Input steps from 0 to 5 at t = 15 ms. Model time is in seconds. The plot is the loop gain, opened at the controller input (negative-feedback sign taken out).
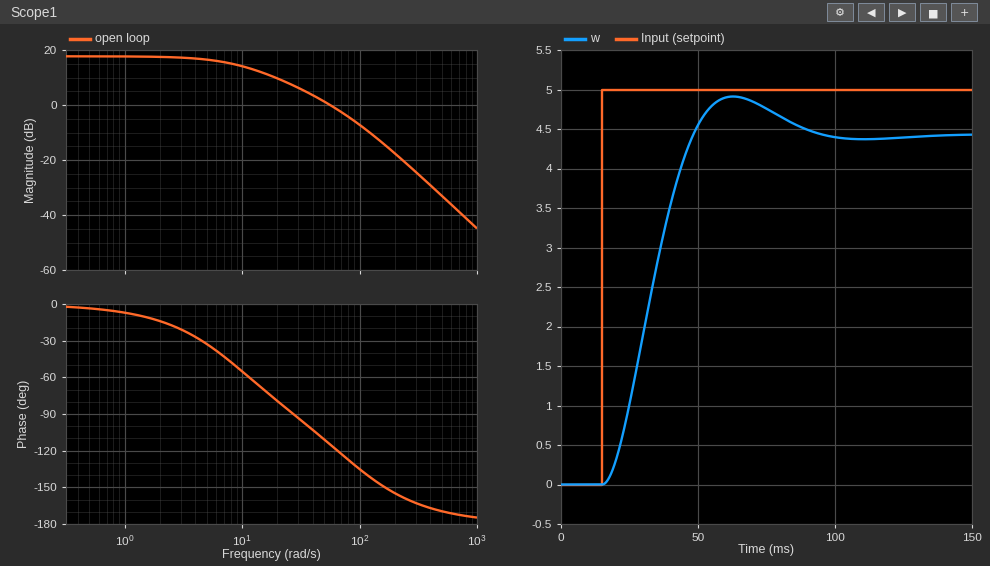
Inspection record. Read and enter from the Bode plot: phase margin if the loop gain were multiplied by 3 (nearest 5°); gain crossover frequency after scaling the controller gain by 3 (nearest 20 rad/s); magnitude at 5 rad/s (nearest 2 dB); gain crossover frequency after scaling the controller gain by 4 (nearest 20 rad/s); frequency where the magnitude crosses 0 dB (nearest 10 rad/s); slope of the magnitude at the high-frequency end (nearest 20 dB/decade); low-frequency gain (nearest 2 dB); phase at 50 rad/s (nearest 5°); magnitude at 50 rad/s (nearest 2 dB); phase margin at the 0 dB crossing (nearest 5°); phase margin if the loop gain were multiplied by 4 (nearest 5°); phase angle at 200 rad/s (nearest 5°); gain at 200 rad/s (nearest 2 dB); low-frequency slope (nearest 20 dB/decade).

40°
120 rad/s
16 dB
140 rad/s
60 rad/s
-40 dB/decade
18 dB
-110°
2 dB
65°
35°
-155°
-18 dB
0 dB/decade
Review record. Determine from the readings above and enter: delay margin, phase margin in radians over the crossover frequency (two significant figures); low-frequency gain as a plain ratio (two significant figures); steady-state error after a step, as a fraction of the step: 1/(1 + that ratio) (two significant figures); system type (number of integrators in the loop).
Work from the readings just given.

0.019 s
7.9
0.11
0
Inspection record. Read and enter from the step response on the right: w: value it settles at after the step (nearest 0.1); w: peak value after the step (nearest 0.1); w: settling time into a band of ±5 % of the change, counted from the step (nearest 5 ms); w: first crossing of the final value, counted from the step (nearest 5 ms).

4.4
4.9
65 ms
35 ms
